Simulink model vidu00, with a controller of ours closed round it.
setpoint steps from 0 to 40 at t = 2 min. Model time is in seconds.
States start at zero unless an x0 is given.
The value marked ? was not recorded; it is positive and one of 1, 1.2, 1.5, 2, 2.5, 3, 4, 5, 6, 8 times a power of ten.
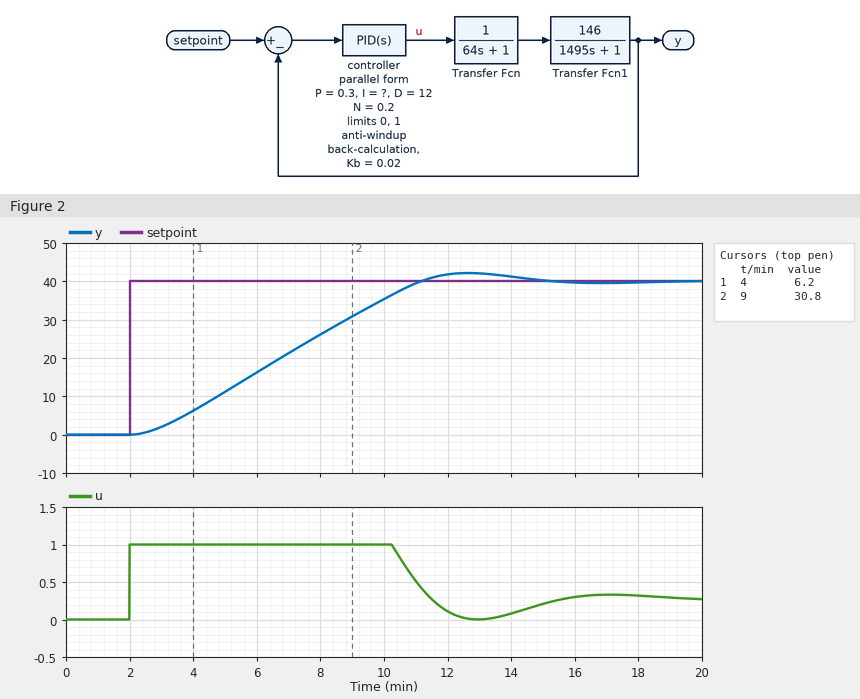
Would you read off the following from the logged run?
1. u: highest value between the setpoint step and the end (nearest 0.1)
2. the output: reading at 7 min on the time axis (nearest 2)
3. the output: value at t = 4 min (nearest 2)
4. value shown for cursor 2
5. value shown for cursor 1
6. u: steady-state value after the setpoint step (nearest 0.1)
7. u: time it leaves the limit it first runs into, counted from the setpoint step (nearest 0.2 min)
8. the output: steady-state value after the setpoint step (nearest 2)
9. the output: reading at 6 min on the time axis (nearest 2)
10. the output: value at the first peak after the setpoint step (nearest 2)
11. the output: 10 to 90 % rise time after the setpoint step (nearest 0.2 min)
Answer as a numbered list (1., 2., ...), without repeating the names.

1. 1.0
2. 22
3. 6
4. 30.8
5. 6.2
6. 0.3
7. 8.2 min
8. 40
9. 16
10. 42
11. 6.6 min
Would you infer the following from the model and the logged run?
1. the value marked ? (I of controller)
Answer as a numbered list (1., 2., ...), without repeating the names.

1. 0.003
